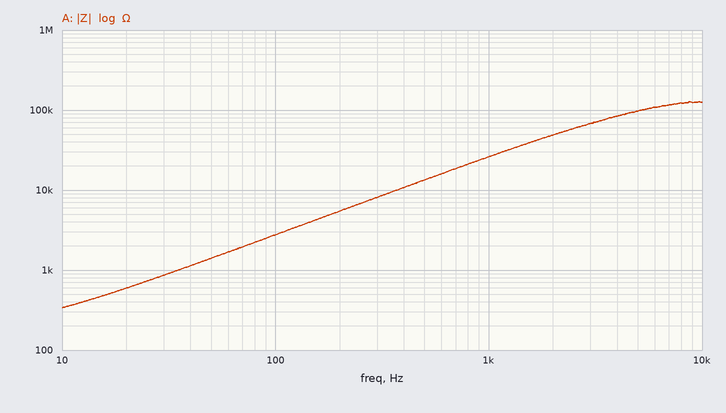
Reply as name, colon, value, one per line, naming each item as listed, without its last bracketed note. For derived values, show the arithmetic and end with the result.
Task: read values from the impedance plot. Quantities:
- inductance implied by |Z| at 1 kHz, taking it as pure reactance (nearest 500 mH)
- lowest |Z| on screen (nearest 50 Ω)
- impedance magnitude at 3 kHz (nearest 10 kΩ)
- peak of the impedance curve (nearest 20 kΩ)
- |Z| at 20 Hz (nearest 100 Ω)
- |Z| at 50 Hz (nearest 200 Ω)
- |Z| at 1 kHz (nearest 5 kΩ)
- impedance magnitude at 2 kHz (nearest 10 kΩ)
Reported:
inductance implied by |Z| at 1 kHz, taking it as pure reactance: L = 25 kΩ/(2π × 1 kHz) ≈ 4.0 H
lowest |Z| on screen: 350 Ω
impedance magnitude at 3 kHz: 70 kΩ
peak of the impedance curve: 120 kΩ
|Z| at 20 Hz: 600 Ω
|Z| at 50 Hz: 1.4 kΩ
|Z| at 1 kHz: 25 kΩ
impedance magnitude at 2 kHz: 50 kΩ
